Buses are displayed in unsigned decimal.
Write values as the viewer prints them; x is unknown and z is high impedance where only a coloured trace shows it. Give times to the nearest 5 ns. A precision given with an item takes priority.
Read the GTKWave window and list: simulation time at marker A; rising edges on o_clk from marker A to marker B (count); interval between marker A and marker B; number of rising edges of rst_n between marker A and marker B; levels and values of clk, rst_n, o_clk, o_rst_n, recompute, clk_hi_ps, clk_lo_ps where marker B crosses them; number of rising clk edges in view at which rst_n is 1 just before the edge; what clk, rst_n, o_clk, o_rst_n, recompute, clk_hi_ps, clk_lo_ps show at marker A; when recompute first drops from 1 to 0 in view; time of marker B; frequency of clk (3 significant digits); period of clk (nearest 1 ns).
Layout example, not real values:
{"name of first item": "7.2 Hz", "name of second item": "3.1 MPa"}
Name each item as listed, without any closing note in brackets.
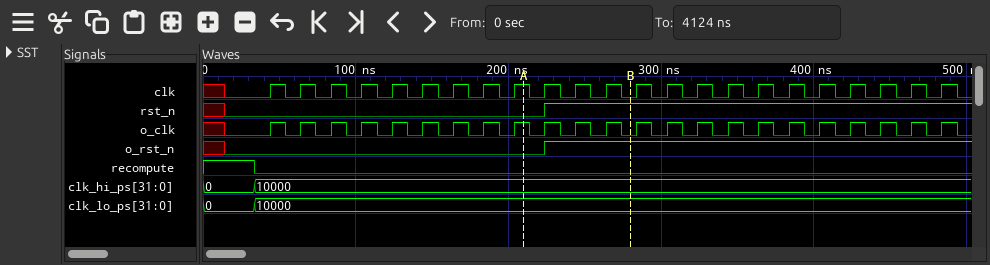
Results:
{"simulation time at marker A": "210 ns", "rising edges on o_clk from marker A to marker B": "3", "interval between marker A and marker B": "70 ns", "number of rising edges of rst_n between marker A and marker B": "1", "levels and values of clk, rst_n, o_clk, o_rst_n, recompute, clk_hi_ps, clk_lo_ps where marker B crosses them": "clk=0, rst_n=1, o_clk=0, o_rst_n=1, recompute=0, clk_hi_ps=10000, clk_lo_ps=10000", "number of rising clk edges in view at which rst_n is 1 just before the edge": "13", "what clk, rst_n, o_clk, o_rst_n, recompute, clk_hi_ps, clk_lo_ps show at marker A": "clk=1, rst_n=0, o_clk=1, o_rst_n=0, recompute=0, clk_hi_ps=10000, clk_lo_ps=10000", "when recompute first drops from 1 to 0 in view": "35 ns", "time of marker B": "280 ns", "frequency of clk": "50.0 MHz", "period of clk": "20 ns"}
